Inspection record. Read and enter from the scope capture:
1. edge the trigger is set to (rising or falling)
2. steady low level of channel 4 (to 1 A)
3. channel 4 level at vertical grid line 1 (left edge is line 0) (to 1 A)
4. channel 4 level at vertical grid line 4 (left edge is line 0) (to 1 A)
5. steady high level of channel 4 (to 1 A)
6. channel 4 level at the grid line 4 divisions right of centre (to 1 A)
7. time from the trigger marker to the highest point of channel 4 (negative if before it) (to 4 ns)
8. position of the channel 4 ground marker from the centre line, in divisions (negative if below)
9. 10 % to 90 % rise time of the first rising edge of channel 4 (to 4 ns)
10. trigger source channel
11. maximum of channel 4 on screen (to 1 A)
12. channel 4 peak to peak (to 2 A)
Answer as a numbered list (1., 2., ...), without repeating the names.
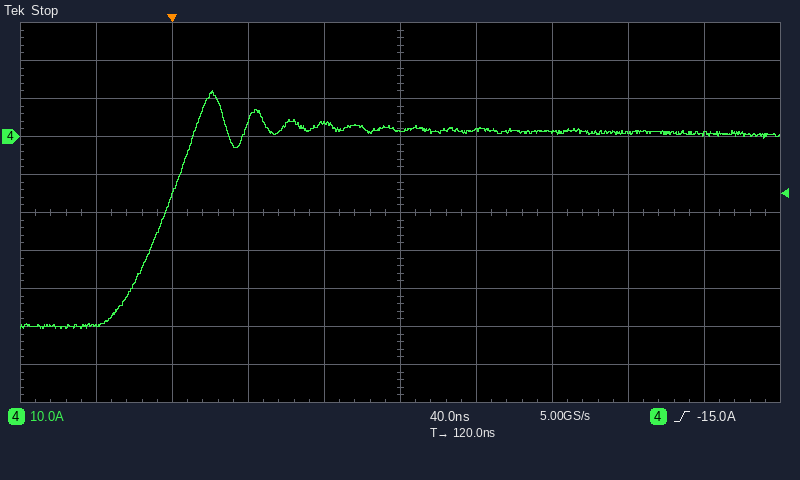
1. rising
2. -50 A
3. -50 A
4. 4 A
5. 1 A
6. 1 A
7. +20 ns
8. +2.0 div
9. 36 ns
10. channel 4
11. 12 A
12. 62 A
